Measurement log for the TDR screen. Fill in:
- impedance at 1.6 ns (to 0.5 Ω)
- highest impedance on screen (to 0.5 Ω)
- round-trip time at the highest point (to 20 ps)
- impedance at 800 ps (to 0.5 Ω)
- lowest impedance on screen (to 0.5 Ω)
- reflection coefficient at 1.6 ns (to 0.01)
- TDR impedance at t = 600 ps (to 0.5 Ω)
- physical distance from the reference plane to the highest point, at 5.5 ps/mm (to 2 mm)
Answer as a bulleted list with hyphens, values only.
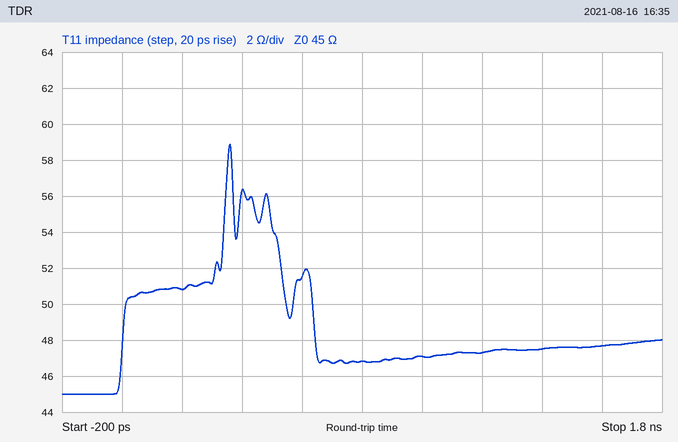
- 47.5 Ω
- 59.0 Ω
- 360 ps
- 47.0 Ω
- 45.0 Ω
- +0.03
- 51.5 Ω
- 32 mm
